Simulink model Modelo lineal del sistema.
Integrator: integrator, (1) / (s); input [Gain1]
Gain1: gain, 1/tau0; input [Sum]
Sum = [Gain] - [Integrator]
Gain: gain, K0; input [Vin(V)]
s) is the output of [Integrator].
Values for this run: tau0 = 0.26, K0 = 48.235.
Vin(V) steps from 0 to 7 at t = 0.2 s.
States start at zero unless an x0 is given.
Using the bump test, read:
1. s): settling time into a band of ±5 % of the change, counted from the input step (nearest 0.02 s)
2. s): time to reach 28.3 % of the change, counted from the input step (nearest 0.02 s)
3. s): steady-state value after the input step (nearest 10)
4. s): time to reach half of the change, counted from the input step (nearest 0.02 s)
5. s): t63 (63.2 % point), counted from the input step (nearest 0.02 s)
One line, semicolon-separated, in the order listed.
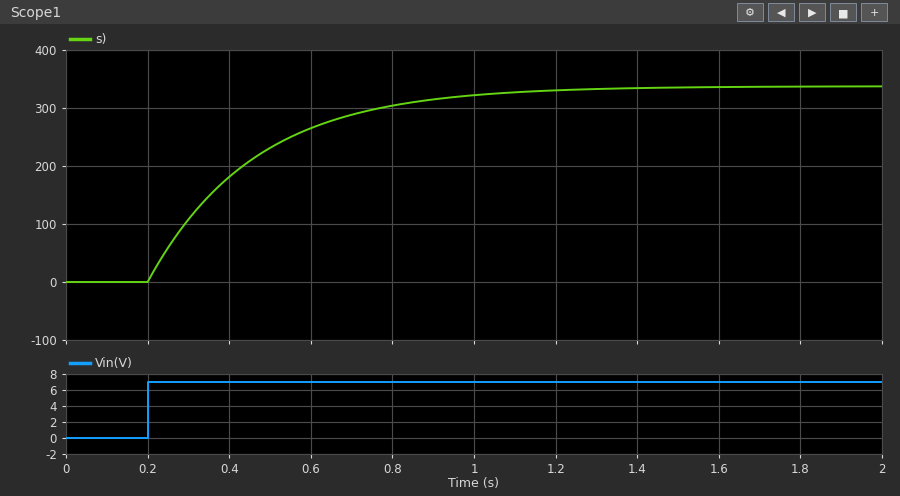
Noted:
0.78 s; 0.08 s; 340; 0.18 s; 0.26 s
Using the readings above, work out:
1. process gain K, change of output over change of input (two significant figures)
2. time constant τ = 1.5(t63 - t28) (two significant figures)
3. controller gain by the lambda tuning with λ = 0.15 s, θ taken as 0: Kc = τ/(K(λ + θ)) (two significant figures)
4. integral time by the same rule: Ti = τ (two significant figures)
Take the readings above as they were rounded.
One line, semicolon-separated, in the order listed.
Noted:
49; 0.27 s; 0.037; 0.27 s
